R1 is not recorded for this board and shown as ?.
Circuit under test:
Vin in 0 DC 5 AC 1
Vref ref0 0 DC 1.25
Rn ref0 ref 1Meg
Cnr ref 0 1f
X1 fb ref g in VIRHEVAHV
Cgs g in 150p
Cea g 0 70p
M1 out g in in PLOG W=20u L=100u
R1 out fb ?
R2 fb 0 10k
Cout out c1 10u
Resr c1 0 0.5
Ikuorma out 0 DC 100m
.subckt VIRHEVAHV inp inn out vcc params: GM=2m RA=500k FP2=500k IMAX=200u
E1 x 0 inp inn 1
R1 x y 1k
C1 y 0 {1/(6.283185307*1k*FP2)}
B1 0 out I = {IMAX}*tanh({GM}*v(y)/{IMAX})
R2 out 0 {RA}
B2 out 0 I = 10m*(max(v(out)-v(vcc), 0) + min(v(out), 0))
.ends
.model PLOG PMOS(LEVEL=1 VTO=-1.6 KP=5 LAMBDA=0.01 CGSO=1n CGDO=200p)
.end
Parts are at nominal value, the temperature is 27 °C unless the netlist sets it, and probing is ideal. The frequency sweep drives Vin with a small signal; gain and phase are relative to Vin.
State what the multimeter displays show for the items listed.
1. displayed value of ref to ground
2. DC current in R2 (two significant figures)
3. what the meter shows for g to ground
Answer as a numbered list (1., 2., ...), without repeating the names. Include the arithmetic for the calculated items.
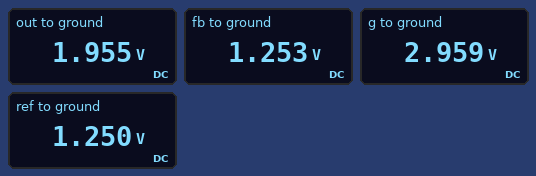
1. 1.250 V
2. (1.253 V) / 10 kΩ = 130 µA
3. 2.959 V
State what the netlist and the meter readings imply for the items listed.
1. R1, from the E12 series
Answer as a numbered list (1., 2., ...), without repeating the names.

1. 5.6 kΩ
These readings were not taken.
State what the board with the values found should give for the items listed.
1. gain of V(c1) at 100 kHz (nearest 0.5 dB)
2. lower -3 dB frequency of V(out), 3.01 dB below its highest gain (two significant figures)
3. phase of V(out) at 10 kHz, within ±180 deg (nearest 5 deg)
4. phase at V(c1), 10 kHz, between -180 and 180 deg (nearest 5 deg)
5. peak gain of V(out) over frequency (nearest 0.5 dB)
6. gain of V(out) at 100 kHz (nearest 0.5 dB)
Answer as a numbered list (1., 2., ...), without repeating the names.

1. -28.5 dB
2. 170 kHz
3. 65 deg
4. 140 deg
5. -20.5 dB
6. -28.0 dB
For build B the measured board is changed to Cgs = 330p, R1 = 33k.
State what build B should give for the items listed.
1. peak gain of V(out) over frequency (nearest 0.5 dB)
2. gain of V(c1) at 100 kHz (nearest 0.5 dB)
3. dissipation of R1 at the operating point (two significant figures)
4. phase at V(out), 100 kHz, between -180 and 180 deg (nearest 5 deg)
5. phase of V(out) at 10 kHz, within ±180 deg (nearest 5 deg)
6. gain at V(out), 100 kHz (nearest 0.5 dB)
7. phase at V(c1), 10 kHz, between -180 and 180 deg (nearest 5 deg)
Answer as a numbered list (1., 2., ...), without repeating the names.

1. 0 dB
2. -4.0 dB
3. 440 µW
4. -5 deg
5. -10 deg
6. -3.5 dB
7. 65 deg
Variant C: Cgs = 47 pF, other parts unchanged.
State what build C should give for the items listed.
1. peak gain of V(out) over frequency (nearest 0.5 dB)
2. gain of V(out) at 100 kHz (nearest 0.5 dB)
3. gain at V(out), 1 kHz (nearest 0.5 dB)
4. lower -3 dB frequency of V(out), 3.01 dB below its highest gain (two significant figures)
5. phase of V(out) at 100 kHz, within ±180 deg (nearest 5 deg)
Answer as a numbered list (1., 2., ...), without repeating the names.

1. -14.0 dB
2. -28.5 dB
3. -56.0 dB
4. 300 kHz
5. 85 deg
